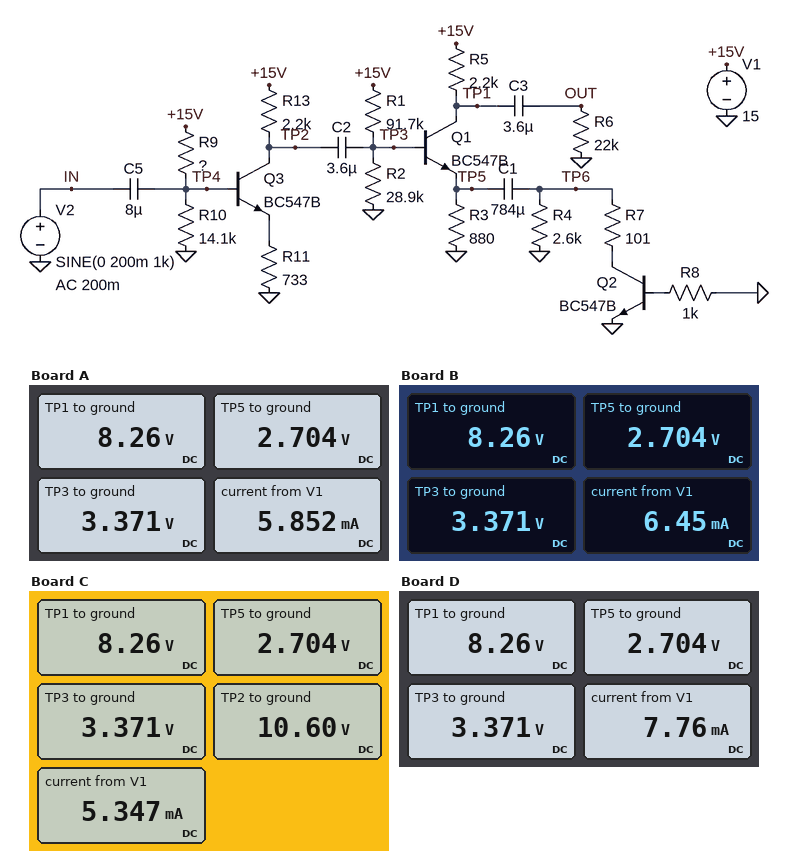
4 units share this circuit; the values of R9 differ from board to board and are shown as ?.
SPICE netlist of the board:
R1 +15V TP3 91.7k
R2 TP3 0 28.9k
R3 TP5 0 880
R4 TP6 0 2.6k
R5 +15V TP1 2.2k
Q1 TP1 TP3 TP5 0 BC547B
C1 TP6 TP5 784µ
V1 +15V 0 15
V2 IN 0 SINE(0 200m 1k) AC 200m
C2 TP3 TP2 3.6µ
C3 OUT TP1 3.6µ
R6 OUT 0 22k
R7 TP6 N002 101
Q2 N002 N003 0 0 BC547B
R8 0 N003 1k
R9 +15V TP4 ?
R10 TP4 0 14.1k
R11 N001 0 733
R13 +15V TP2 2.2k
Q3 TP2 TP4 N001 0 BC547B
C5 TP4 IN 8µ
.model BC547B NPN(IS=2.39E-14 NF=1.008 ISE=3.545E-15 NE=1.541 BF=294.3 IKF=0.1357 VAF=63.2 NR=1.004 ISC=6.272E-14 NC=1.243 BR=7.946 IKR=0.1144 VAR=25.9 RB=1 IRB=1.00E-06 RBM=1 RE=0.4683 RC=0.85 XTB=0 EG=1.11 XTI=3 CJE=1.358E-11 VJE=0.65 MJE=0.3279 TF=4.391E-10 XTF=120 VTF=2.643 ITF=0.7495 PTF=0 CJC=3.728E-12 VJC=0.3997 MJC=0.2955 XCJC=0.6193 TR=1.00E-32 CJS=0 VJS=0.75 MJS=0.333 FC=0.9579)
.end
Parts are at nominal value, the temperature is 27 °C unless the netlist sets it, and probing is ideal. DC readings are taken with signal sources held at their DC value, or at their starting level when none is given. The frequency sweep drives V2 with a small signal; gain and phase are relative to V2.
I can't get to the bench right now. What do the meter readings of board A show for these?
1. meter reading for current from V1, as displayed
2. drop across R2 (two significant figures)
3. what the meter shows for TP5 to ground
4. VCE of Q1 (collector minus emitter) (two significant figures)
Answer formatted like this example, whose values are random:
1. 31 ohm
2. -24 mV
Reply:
1. 5.852 mA
2. 3.4 V
3. 2.704 V
4. 5.6 V
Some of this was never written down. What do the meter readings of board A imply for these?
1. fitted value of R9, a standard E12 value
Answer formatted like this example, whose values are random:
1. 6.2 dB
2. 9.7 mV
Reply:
1. 68 kΩ
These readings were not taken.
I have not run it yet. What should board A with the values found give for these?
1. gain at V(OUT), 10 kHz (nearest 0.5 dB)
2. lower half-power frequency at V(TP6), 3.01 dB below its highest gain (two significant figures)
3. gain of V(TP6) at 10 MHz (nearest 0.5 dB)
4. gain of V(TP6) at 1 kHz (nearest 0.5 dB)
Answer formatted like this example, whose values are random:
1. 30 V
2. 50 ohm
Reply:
1. 18.0 dB
2. 3.0 Hz
3. 4.0 dB
4. 8.5 dB
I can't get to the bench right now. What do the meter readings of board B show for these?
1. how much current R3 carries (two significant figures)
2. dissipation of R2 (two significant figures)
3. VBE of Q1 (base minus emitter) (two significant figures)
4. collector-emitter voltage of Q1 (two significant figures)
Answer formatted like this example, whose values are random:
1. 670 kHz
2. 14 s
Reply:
1. 3.1 mA
2. 390 µW
3. 670 mV
4. 5.6 V
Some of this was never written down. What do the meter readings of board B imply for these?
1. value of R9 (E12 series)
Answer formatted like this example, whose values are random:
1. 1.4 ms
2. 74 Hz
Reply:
1. 56 kΩ
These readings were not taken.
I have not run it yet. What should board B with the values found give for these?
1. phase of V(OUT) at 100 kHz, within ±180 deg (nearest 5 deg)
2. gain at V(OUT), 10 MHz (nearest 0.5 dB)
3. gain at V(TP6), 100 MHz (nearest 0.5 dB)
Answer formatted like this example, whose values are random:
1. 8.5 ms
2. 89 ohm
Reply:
1. 0 deg
2. 13.5 dB
3. -7.0 dB
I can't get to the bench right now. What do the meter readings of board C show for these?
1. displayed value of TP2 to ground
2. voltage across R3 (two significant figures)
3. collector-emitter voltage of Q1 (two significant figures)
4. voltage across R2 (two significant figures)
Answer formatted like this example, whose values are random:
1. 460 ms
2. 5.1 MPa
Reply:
1. 10.60 V
2. 2.7 V
3. 5.6 V
4. 3.4 V
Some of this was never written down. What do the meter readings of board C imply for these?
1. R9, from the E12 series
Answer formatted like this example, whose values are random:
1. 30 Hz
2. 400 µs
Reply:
1. 82 kΩ
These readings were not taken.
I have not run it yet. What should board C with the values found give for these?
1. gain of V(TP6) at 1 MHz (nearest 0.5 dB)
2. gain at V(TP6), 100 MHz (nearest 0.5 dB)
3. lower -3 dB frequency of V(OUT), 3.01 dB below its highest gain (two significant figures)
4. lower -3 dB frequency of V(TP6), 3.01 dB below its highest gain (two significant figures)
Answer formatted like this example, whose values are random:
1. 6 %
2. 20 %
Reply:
1. 8.0 dB
2. -7.5 dB
3. 3.7 Hz
4. 2.9 Hz
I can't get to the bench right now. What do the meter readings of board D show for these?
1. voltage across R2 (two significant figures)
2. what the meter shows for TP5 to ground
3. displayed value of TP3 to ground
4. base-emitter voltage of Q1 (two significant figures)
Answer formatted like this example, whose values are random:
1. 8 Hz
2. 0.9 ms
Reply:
1. 3.4 V
2. 2.704 V
3. 3.371 V
4. 670 mV
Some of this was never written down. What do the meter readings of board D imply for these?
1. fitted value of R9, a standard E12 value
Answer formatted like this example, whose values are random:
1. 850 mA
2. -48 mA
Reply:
1. 39 kΩ
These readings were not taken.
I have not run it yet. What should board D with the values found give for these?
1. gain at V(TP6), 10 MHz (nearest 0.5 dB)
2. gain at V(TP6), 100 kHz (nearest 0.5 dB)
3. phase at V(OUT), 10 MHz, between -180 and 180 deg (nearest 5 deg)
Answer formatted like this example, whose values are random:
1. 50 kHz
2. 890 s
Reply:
1. 3.5 dB
2. 8.5 dB
3. -70 deg
